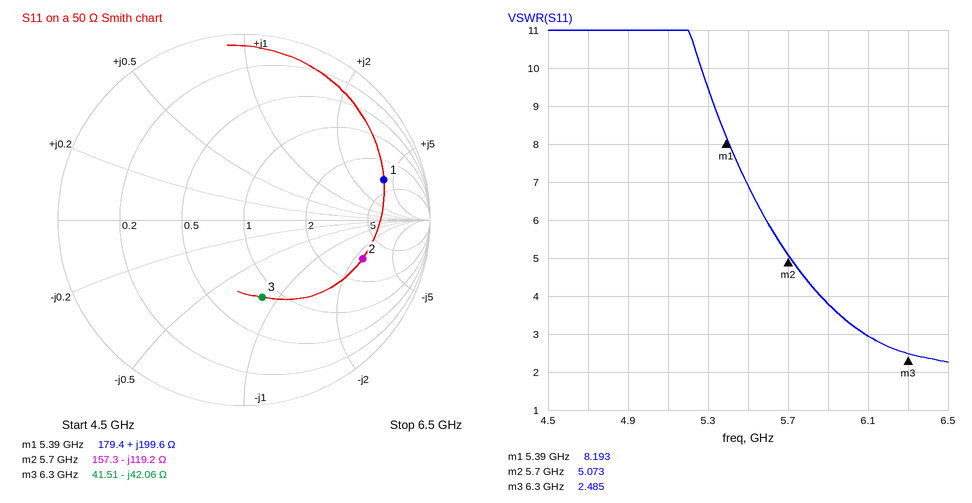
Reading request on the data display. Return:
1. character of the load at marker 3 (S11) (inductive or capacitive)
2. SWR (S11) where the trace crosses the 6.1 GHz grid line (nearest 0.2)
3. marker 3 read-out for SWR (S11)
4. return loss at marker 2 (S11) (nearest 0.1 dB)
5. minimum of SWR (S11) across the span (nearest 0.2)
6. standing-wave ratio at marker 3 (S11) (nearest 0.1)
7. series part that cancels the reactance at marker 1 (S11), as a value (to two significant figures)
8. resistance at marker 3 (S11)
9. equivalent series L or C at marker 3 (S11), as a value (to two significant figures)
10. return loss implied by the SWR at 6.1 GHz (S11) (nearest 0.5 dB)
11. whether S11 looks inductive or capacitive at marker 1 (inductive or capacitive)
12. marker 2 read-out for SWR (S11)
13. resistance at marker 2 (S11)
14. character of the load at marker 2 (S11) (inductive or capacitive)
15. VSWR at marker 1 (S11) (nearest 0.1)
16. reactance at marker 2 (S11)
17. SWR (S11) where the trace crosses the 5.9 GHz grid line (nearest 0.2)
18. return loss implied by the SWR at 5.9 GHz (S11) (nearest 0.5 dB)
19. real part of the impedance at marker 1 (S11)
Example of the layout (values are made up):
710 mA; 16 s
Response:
capacitive; 3.0; 2.485; 3.5 dB; 2.2; 2.5; 150 fF; 41.51 Ω; 600 fF; 6.0 dB; inductive; 5.073; 157.3 Ω; capacitive; 8.2; -119.2 Ω; 3.8; 4.5 dB; 179.4 Ω
